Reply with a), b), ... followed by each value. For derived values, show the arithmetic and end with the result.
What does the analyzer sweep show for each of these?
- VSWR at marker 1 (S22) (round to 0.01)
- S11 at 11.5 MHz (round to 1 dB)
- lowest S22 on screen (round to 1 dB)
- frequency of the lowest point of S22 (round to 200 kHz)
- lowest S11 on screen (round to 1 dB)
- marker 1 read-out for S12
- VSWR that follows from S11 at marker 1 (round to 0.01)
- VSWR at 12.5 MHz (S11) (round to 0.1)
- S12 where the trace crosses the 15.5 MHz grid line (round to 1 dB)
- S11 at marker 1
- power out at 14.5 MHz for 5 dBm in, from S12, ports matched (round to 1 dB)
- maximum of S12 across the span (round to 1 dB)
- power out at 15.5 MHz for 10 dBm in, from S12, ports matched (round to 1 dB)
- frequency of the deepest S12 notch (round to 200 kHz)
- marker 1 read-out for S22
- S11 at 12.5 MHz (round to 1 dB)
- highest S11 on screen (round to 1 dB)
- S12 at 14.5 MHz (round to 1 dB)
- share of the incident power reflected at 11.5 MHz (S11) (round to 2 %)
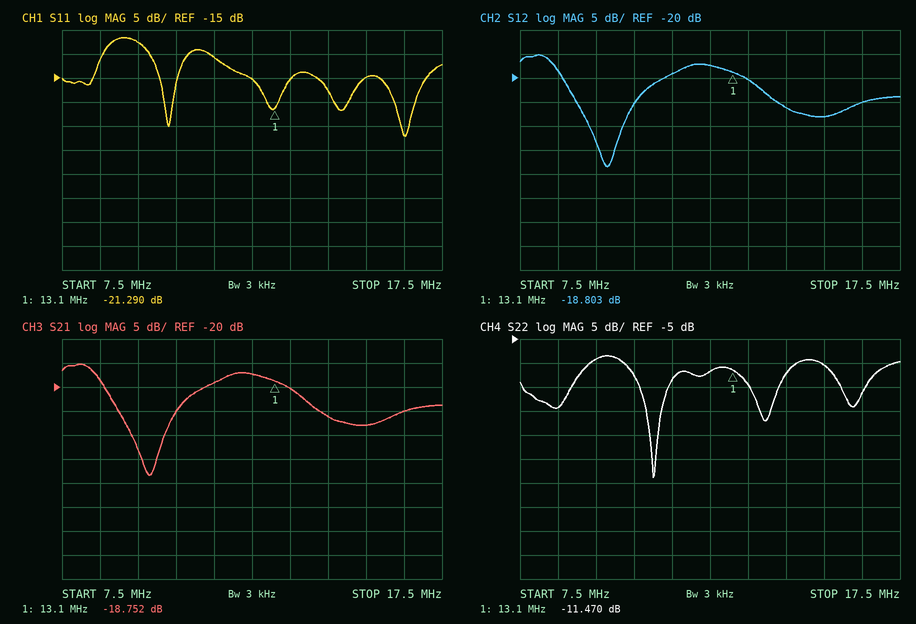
a) (1 + 0.2670)/(1 − 0.2670) ≈ 1.73
b) -11 dB
c) -34 dB
d) 11.0 MHz
e) -27 dB
f) -18.803 dB
g) (1 + 0.0862)/(1 − 0.0862) ≈ 1.19
h) |Γ| = 10^(-15/20) = 0.1778; VSWR = (1 + 0.1778)/(1 − 0.1778) ≈ 1.4
i) -28 dB
j) -21.290 dB
k) 5 dBm + (-26 dB) = -21 dBm
l) -15 dB
m) 10 dBm + (-28 dB) = -18 dBm
n) 9.8 MHz
o) -11.470 dB
p) -15 dB
q) -7 dB
r) -26 dB
s) 10^(-11/10) ≈ 8 %
